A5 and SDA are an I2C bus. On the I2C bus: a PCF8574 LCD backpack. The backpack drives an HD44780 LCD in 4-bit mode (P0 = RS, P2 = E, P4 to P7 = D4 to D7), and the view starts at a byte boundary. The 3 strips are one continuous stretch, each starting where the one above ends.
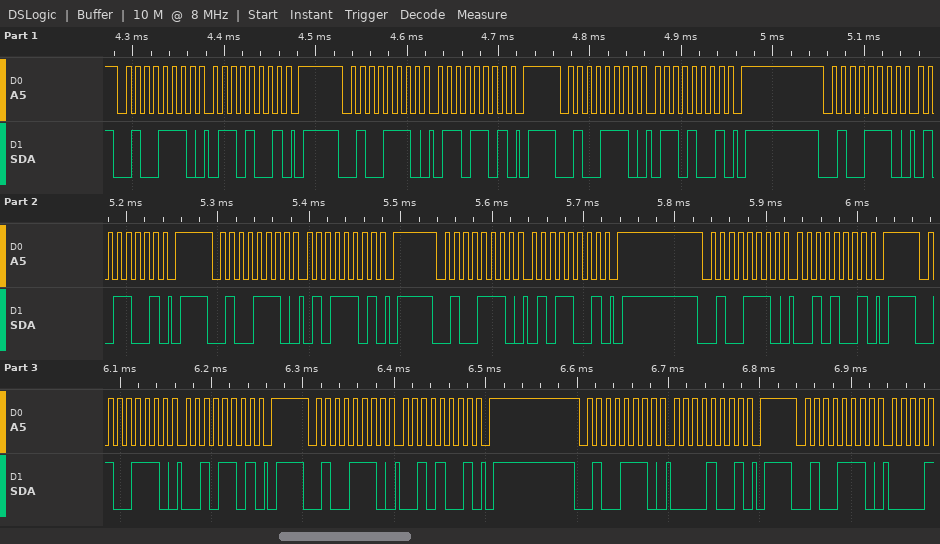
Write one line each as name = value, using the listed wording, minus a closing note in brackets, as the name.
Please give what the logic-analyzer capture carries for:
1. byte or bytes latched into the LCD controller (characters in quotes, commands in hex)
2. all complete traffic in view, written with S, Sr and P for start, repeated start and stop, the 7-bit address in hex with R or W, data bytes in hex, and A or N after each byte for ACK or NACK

byte or bytes latched into the LCD controller = 'e'
all complete traffic in view, written with S, Sr and P for start, repeated start and stop, the 7-bit address in hex with R or W, data bytes in hex, and A or N after each byte for ACK or NACK = S 27W A 69 A P S 27W A 6D A P S 27W A 69 A P S 27W A 59 A P S 27W A 5D A P S 27W A 59 A P S 27W A 29 A P S 27W A 2D A P S 27W A 29 A P S 27W A 09 A P S 27W A
